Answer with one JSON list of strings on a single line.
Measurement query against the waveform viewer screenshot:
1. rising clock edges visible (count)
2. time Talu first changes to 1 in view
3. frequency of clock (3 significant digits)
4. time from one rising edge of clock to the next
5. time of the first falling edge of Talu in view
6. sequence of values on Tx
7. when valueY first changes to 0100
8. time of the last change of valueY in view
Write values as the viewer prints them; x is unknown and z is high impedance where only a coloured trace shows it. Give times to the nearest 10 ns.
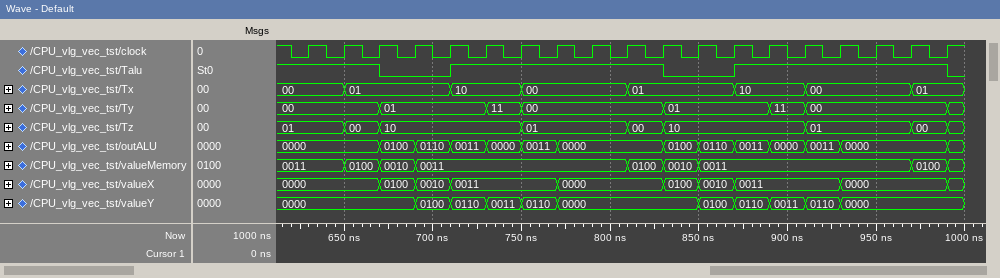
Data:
["19", "710 ns", "50.0 MHz", "20 ns", "670 ns", "00, 01, 10, 00, 01, 10, 00, 01", "690 ns", "930 ns"]
